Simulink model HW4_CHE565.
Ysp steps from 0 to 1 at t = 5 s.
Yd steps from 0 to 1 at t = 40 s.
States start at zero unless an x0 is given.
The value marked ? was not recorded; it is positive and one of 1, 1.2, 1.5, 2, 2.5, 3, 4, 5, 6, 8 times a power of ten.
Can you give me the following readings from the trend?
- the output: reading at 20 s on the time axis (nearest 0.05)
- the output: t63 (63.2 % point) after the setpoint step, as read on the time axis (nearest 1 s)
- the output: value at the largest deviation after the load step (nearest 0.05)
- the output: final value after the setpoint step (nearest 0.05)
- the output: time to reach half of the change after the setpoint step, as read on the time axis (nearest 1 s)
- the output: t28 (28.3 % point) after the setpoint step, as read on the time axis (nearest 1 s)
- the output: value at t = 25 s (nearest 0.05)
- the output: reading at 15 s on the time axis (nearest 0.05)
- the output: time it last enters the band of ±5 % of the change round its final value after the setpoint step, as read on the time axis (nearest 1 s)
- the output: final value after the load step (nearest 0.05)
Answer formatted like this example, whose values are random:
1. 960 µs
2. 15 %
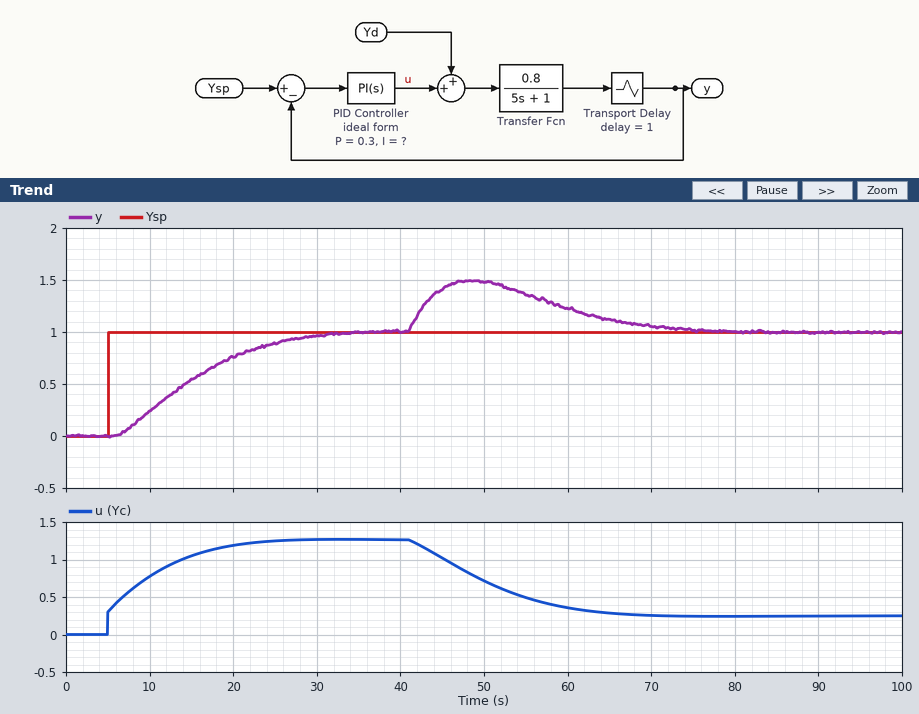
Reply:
1. 0.75
2. 17 s
3. 1.50
4. 1.00
5. 14 s
6. 11 s
7. 0.90
8. 0.55
9. 29 s
10. 1.00
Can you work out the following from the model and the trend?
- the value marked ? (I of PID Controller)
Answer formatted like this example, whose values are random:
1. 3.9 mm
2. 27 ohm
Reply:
1. 0.4
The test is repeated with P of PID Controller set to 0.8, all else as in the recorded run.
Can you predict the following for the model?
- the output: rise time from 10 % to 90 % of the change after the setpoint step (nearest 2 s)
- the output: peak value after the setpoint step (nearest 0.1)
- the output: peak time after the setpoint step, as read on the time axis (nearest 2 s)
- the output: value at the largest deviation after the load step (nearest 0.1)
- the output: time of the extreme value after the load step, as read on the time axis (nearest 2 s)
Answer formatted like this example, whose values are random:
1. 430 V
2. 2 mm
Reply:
1. 6 s
2. 1.1
3. 20 s
4. 1.4
5. 46 s
